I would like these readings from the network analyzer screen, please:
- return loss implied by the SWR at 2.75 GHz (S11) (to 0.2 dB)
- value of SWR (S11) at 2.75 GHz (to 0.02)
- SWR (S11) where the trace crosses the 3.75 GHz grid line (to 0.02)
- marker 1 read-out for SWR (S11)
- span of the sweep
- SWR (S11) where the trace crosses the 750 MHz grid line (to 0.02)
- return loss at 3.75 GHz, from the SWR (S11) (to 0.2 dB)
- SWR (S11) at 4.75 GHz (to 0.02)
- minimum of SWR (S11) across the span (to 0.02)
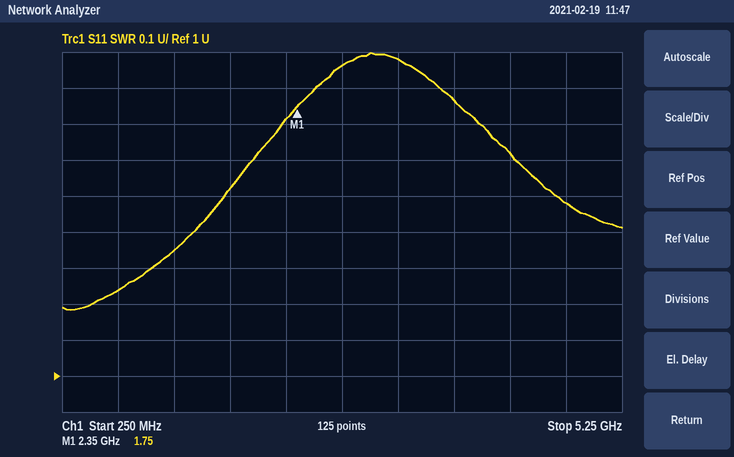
10.4 dB
1.86
1.76
1.75
5 GHz
1.24
11.2 dB
1.48
1.18
